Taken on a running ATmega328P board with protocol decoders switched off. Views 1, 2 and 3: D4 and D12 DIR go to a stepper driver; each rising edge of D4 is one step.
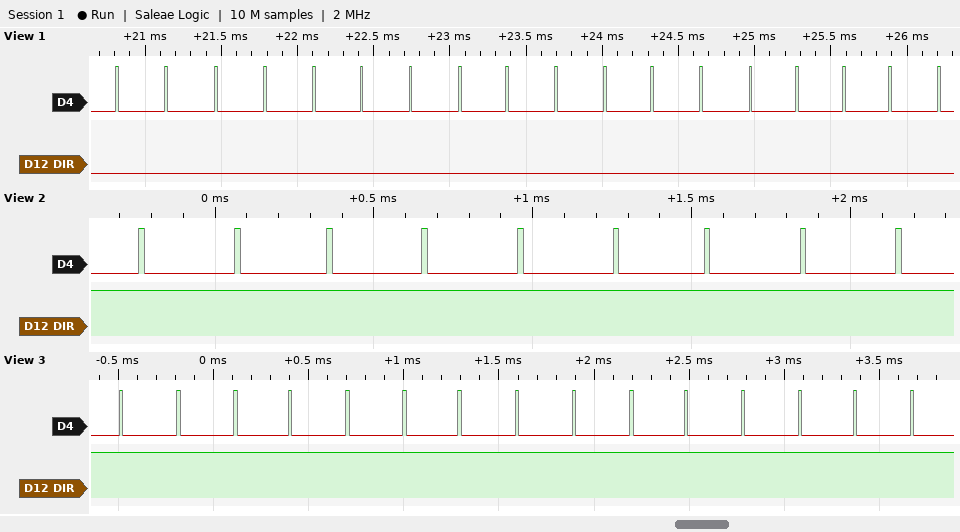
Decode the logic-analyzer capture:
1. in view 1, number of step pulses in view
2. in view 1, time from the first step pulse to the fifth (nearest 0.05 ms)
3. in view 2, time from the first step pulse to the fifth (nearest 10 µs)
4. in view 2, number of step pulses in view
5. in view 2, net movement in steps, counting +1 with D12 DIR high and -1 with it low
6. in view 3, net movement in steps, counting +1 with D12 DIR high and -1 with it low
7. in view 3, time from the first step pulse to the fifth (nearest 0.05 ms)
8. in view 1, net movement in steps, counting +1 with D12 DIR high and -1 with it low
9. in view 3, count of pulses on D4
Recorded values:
18
1.30 ms
1190 µs
9
+9
+15
1.20 ms
-18
15
